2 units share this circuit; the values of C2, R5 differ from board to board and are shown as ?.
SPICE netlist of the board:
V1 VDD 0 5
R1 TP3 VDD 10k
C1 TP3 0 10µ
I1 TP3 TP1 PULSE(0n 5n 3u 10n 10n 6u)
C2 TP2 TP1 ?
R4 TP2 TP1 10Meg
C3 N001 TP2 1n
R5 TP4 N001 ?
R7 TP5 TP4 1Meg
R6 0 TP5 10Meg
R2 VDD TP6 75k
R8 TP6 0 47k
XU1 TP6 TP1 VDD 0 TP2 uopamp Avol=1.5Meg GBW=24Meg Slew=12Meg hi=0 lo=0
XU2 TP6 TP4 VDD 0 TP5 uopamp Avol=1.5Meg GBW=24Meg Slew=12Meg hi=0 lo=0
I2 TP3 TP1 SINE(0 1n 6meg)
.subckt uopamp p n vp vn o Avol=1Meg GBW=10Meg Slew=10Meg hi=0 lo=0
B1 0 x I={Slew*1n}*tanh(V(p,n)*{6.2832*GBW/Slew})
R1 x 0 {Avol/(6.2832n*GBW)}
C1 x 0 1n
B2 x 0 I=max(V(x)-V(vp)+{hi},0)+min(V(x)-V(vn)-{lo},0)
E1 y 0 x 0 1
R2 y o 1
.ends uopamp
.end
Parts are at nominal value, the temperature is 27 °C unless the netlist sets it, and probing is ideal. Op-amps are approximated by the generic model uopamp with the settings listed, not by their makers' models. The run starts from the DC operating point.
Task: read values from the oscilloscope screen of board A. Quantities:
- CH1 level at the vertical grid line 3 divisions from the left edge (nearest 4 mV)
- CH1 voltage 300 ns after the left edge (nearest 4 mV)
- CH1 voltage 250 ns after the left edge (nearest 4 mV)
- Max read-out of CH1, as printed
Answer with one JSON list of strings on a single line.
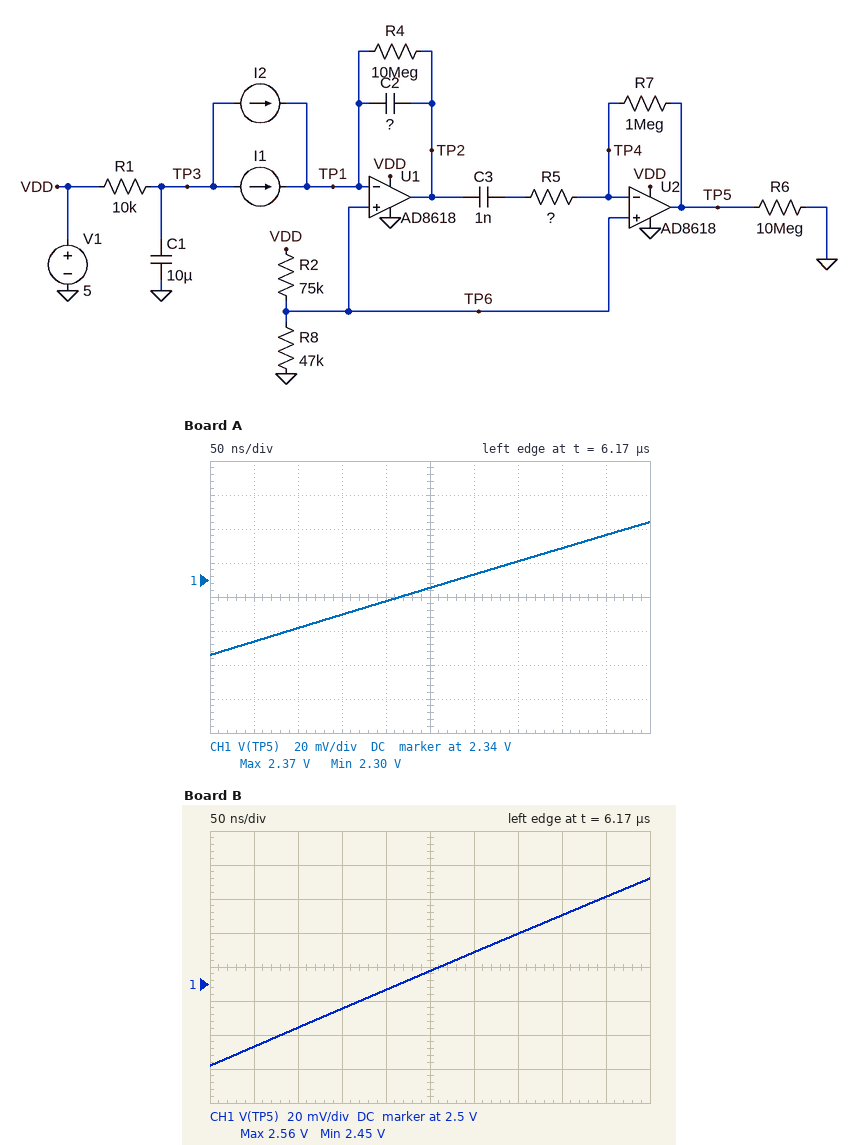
["2.320 V", "2.344 V", "2.336 V", "2.37 V"]
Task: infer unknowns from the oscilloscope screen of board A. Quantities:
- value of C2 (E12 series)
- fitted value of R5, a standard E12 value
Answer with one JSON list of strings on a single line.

["5.6 pF", "3.3 kΩ"]
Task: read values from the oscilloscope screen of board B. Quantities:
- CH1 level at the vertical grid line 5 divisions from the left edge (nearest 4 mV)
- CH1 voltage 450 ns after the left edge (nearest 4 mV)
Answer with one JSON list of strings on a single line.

["2.508 V", "2.552 V"]
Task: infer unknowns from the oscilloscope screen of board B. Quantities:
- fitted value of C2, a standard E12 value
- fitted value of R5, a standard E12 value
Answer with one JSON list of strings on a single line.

["3.9 pF", "3.3 kΩ"]
